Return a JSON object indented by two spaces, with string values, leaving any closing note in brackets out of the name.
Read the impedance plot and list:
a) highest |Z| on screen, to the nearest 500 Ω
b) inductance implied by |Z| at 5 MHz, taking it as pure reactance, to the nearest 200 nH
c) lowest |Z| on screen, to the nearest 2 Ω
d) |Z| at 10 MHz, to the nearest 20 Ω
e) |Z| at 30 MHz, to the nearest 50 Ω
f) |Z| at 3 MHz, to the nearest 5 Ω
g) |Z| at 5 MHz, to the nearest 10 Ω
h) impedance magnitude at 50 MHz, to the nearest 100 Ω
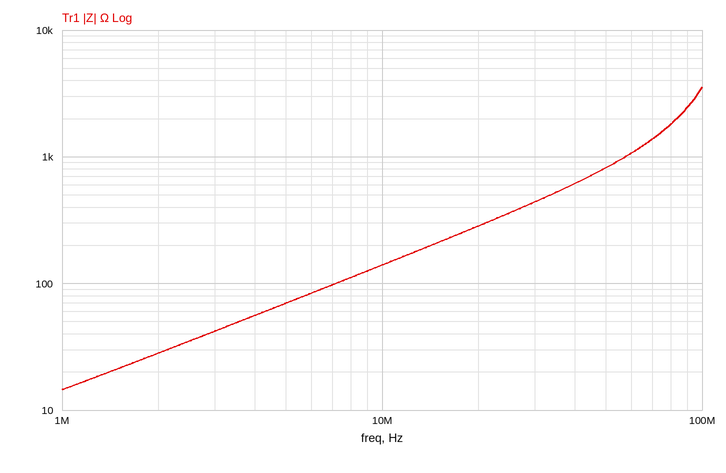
{
  "highest |Z| on screen, to the nearest 500 Ω": "3.5 kΩ",
  "inductance implied by |Z| at 5 MHz, taking it as pure reactance, to the nearest 200 nH": "2.2 µH",
  "lowest |Z| on screen, to the nearest 2 Ω": "14 Ω",
  "|Z| at 10 MHz, to the nearest 20 Ω": "140 Ω",
  "|Z| at 30 MHz, to the nearest 50 Ω": "450 Ω",
  "|Z| at 3 MHz, to the nearest 5 Ω": "40 Ω",
  "|Z| at 5 MHz, to the nearest 10 Ω": "70 Ω",
  "impedance magnitude at 50 MHz, to the nearest 100 Ω": "800 Ω"
}
